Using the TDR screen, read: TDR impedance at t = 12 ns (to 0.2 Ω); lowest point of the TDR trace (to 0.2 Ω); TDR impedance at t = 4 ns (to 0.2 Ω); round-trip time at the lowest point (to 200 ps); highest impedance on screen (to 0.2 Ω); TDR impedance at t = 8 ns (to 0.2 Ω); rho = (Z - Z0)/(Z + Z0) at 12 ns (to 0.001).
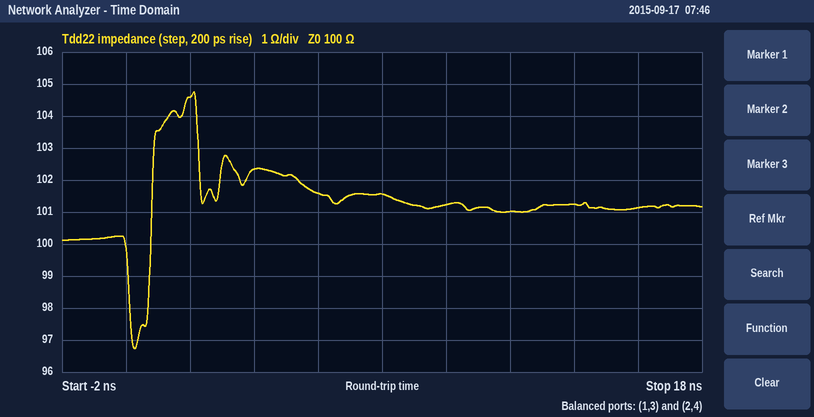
101.0 Ω
96.8 Ω
102.4 Ω
200 ps
104.8 Ω
101.6 Ω
+0.005
